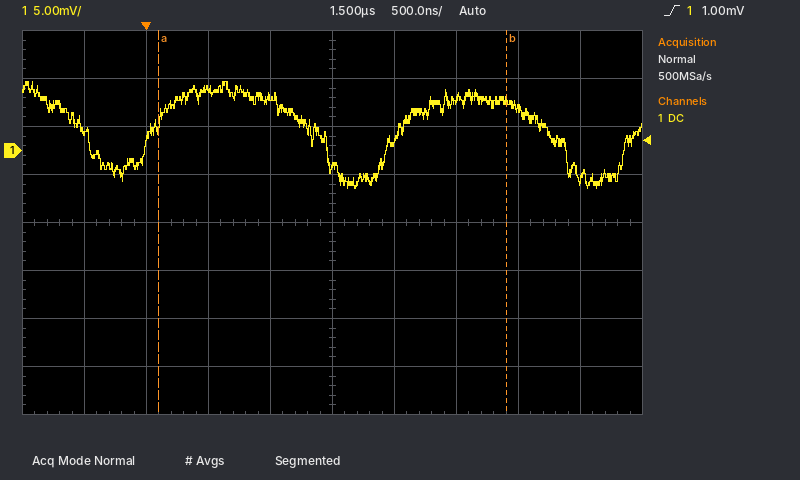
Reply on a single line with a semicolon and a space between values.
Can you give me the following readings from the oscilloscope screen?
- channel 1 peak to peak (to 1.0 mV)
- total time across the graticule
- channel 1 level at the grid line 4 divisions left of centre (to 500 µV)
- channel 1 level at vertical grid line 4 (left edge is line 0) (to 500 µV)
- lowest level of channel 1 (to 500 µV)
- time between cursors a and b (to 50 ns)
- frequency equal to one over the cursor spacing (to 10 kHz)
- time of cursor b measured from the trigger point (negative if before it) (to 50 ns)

11.0 mV; 5 µs; 2.0 mV; 5.5 mV; -4.0 mV; 2.80 µs; 360 kHz; +2.90 µs
